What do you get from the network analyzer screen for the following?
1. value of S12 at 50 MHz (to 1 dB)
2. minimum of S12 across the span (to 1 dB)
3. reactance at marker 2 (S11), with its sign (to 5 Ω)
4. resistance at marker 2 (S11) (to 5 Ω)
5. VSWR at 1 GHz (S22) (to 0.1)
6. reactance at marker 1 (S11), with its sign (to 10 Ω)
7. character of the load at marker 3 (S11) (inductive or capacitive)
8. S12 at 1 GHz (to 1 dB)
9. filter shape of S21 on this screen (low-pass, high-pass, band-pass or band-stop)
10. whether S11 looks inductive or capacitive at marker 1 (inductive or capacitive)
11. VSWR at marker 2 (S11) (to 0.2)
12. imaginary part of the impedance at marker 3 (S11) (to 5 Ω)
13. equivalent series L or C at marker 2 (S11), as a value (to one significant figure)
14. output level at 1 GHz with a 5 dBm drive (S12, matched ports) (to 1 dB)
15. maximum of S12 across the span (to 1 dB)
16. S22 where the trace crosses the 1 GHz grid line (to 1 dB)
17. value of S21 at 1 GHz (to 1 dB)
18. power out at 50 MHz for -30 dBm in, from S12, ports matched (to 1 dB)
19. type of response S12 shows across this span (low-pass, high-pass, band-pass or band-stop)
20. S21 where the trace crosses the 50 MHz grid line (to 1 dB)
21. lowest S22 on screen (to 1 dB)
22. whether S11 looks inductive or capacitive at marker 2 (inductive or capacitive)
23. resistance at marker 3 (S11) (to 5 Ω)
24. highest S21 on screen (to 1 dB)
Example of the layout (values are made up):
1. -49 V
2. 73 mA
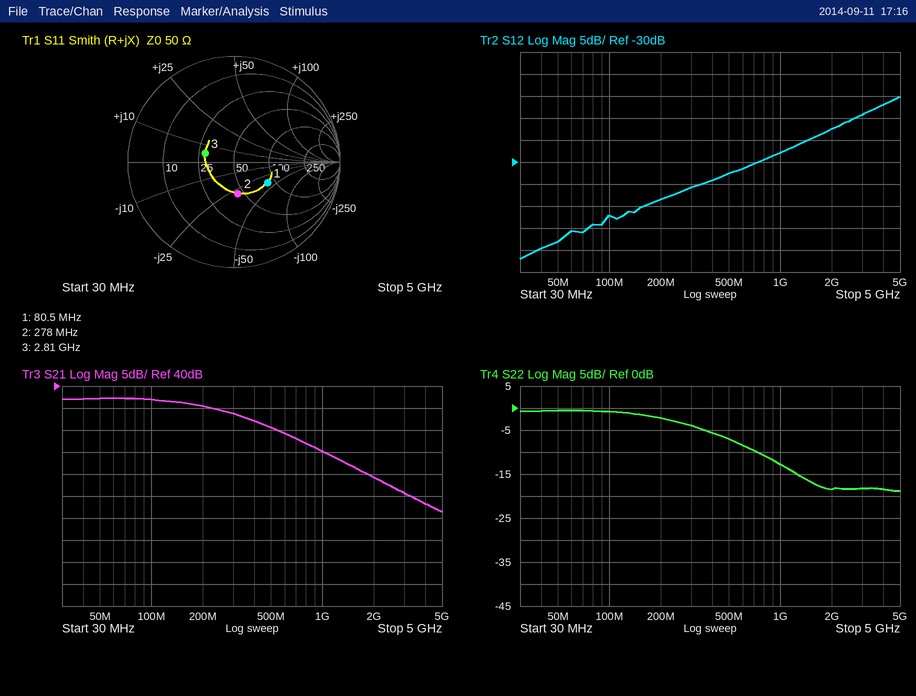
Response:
1. -48 dB
2. -52 dB
3. -30 Ω
4. 45 Ω
5. 1.6
6. -40 Ω
7. inductive
8. -28 dB
9. low-pass
10. capacitive
11. 1.8
12. +5 Ω
13. 20 pF
14. -23 dBm
15. -15 dB
16. -13 dB
17. 25 dB
18. -78 dBm
19. high-pass
20. 37 dB
21. -19 dB
22. capacitive
23. 30 Ω
24. 37 dB
